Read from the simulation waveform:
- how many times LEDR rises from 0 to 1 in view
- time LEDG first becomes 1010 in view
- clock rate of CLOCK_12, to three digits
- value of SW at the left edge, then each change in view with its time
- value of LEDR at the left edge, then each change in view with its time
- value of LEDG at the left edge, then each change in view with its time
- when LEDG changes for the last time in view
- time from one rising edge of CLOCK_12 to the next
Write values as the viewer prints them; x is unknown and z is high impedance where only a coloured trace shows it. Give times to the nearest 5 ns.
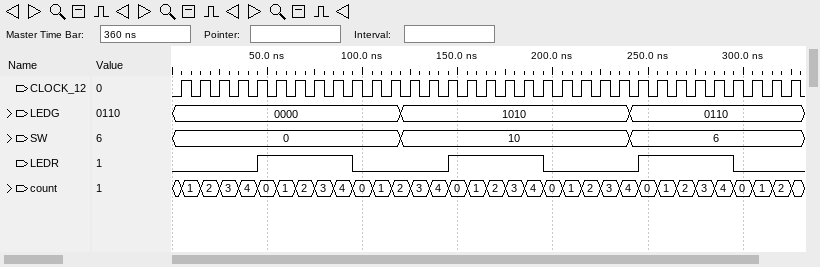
3
120 ns
100 MHz
0, 10 at 120 ns, 6 at 240 ns
0, 1 at 45 ns, 0 at 95 ns, 1 at 145 ns, 0 at 195 ns, 1 at 245 ns, 0 at 295 ns
0000, 1010 at 120 ns, 0110 at 240 ns
240 ns
10 ns
